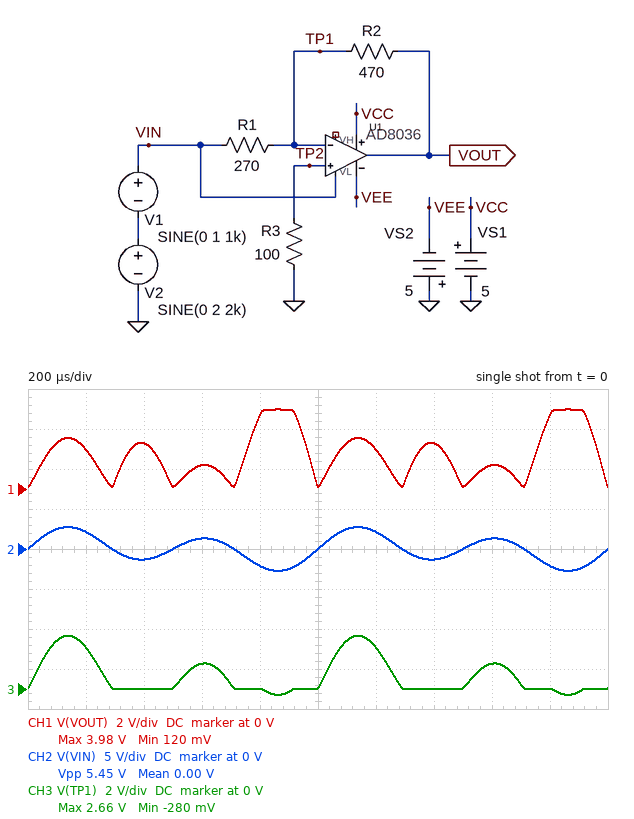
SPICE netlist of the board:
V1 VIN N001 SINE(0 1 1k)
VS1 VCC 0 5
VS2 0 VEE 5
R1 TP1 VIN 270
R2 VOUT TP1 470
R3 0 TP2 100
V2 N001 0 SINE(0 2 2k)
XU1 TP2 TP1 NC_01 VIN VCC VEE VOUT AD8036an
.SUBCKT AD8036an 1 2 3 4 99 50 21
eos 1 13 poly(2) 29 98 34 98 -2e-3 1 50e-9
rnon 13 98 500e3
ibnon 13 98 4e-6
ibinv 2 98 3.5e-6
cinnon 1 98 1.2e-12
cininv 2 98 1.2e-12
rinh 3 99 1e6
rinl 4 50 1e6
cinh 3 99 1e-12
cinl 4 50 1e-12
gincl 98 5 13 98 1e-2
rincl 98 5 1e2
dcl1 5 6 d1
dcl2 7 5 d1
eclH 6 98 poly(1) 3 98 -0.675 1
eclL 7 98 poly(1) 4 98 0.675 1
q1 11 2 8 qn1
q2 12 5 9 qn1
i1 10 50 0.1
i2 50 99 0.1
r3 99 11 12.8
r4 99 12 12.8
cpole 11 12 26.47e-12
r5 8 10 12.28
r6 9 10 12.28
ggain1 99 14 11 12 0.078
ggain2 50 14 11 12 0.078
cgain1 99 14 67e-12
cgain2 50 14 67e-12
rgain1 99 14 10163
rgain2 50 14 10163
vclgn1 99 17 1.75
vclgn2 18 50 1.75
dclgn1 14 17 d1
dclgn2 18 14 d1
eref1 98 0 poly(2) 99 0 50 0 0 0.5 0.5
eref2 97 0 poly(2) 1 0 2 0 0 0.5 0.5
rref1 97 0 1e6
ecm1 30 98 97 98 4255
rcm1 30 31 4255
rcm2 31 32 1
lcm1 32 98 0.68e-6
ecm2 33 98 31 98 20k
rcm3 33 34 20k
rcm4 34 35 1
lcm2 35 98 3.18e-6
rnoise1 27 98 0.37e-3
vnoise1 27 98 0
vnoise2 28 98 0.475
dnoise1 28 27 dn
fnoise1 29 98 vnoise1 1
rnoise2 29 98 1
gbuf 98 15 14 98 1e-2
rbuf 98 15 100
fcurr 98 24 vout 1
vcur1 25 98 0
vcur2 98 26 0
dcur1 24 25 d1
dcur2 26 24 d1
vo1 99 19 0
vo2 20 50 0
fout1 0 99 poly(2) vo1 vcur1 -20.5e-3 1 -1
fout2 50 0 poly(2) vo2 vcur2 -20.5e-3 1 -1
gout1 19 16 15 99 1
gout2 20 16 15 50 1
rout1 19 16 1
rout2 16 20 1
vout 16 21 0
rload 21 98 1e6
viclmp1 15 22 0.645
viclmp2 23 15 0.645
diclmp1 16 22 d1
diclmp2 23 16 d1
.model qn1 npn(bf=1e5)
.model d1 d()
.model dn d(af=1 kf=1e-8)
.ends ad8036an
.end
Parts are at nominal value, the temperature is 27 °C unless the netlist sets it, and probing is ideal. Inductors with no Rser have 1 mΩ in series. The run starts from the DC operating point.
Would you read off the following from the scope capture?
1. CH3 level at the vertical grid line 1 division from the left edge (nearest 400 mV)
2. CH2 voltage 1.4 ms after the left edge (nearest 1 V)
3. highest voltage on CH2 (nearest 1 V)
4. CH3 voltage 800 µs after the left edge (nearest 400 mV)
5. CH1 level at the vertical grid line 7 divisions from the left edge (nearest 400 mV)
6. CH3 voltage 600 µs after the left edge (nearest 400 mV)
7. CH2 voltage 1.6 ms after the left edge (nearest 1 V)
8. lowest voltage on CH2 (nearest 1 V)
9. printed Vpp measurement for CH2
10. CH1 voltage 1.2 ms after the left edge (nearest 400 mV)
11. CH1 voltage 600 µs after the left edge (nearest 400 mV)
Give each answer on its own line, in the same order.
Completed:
2.0 V
-1 V
3 V
0 V
2.4 V
1.2 V
1 V
-3 V
5.45 V
2.0 V
1.2 V
